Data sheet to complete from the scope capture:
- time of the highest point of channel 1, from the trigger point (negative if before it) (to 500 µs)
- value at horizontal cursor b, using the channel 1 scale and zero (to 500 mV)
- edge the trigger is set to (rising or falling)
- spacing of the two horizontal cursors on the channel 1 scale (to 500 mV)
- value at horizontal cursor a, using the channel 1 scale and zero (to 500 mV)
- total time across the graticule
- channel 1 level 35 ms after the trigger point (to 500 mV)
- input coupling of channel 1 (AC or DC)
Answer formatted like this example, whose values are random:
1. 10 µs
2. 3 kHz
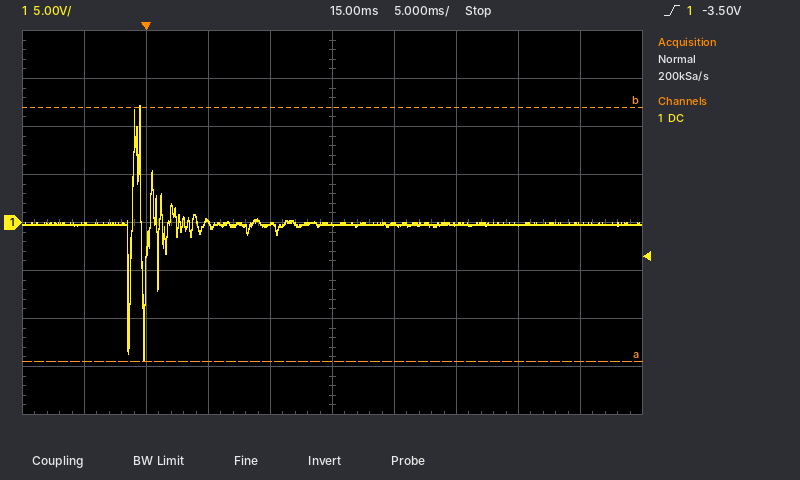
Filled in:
1. -500 µs
2. 12.0 V
3. rising
4. 26.5 V
5. -14.5 V
6. 50 ms
7. 0.0 V
8. DC
